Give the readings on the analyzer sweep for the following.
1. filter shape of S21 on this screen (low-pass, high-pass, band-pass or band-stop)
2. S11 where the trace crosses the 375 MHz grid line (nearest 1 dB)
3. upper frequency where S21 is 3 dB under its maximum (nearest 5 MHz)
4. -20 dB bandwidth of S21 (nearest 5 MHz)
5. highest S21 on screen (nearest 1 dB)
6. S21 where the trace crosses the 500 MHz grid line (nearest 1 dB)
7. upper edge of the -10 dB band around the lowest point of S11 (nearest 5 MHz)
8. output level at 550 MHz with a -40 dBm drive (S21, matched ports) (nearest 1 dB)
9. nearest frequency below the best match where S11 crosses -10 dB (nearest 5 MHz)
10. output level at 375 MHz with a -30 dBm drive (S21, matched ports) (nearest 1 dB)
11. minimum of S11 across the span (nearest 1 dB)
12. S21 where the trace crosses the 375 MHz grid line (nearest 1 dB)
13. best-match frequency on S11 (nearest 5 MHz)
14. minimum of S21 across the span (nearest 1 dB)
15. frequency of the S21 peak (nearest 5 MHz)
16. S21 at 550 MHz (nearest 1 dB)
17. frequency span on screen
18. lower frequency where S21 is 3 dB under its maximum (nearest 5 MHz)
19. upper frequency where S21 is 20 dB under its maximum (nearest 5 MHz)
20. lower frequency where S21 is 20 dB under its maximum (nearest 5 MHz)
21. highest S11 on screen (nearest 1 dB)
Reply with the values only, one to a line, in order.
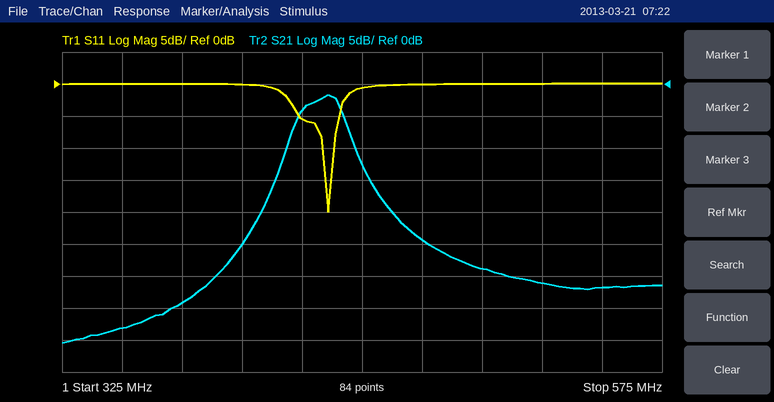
band-pass
0 dB
440 MHz
60 MHz
-2 dB
-29 dB
440 MHz
-72 dBm
435 MHz
-64 dBm
-20 dB
-34 dB
435 MHz
-40 dB
435 MHz
-32 dB
250 MHz
425 MHz
465 MHz
405 MHz
0 dB
